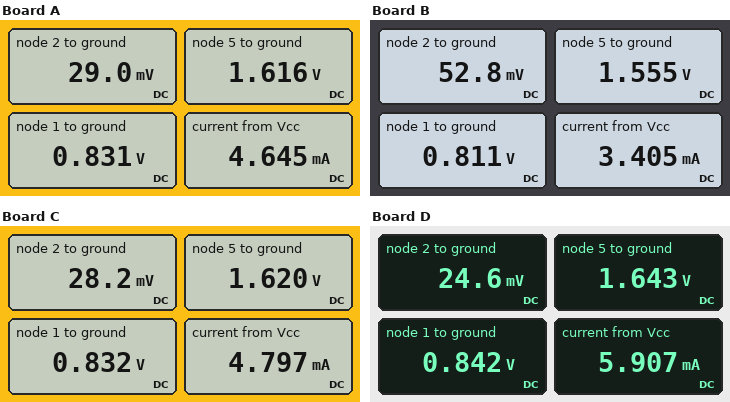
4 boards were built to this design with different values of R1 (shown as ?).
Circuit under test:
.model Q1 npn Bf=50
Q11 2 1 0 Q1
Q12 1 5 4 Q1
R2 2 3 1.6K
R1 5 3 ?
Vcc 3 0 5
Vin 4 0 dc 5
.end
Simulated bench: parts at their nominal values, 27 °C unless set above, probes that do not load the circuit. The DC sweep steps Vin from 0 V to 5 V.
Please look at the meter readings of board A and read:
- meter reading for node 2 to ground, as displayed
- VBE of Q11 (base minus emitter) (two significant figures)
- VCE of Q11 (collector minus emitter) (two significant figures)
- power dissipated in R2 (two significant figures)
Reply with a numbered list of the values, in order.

1. 29.0 mV
2. 830 mV
3. 29 mV
4. 15 mW
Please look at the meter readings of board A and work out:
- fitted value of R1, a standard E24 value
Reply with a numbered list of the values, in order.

1. 2.2 kΩ
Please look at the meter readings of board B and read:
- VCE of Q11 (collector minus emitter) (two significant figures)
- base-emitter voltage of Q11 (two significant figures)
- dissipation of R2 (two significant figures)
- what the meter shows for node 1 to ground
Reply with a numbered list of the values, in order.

1. 53 mV
2. 810 mV
3. 15 mW
4. 0.811 V
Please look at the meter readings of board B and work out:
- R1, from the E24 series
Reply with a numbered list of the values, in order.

1. 11 kΩ
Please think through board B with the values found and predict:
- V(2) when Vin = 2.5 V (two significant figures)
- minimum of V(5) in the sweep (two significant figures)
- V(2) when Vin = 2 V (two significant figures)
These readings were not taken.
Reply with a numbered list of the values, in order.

1. 53 mV
2. 770 mV
3. 53 mV
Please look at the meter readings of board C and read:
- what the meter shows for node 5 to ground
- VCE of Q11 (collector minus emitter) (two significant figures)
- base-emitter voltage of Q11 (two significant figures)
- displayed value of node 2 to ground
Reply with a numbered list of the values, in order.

1. 1.620 V
2. 28 mV
3. 830 mV
4. 28.2 mV
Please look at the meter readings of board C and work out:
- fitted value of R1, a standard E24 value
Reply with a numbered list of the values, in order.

1. 2 kΩ
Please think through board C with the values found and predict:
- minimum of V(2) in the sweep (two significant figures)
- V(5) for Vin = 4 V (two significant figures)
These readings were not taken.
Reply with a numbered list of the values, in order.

1. 28 mV
2. 1.6 V
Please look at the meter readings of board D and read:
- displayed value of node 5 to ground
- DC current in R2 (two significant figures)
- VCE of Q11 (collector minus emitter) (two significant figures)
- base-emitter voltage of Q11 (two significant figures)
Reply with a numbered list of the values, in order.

1. 1.643 V
2. 3.1 mA
3. 25 mV
4. 840 mV
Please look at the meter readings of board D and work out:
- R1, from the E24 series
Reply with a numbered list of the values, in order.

1. 1.2 kΩ
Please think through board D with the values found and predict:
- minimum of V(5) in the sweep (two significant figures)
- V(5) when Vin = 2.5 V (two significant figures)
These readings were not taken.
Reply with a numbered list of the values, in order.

1. 820 mV
2. 1.6 V
